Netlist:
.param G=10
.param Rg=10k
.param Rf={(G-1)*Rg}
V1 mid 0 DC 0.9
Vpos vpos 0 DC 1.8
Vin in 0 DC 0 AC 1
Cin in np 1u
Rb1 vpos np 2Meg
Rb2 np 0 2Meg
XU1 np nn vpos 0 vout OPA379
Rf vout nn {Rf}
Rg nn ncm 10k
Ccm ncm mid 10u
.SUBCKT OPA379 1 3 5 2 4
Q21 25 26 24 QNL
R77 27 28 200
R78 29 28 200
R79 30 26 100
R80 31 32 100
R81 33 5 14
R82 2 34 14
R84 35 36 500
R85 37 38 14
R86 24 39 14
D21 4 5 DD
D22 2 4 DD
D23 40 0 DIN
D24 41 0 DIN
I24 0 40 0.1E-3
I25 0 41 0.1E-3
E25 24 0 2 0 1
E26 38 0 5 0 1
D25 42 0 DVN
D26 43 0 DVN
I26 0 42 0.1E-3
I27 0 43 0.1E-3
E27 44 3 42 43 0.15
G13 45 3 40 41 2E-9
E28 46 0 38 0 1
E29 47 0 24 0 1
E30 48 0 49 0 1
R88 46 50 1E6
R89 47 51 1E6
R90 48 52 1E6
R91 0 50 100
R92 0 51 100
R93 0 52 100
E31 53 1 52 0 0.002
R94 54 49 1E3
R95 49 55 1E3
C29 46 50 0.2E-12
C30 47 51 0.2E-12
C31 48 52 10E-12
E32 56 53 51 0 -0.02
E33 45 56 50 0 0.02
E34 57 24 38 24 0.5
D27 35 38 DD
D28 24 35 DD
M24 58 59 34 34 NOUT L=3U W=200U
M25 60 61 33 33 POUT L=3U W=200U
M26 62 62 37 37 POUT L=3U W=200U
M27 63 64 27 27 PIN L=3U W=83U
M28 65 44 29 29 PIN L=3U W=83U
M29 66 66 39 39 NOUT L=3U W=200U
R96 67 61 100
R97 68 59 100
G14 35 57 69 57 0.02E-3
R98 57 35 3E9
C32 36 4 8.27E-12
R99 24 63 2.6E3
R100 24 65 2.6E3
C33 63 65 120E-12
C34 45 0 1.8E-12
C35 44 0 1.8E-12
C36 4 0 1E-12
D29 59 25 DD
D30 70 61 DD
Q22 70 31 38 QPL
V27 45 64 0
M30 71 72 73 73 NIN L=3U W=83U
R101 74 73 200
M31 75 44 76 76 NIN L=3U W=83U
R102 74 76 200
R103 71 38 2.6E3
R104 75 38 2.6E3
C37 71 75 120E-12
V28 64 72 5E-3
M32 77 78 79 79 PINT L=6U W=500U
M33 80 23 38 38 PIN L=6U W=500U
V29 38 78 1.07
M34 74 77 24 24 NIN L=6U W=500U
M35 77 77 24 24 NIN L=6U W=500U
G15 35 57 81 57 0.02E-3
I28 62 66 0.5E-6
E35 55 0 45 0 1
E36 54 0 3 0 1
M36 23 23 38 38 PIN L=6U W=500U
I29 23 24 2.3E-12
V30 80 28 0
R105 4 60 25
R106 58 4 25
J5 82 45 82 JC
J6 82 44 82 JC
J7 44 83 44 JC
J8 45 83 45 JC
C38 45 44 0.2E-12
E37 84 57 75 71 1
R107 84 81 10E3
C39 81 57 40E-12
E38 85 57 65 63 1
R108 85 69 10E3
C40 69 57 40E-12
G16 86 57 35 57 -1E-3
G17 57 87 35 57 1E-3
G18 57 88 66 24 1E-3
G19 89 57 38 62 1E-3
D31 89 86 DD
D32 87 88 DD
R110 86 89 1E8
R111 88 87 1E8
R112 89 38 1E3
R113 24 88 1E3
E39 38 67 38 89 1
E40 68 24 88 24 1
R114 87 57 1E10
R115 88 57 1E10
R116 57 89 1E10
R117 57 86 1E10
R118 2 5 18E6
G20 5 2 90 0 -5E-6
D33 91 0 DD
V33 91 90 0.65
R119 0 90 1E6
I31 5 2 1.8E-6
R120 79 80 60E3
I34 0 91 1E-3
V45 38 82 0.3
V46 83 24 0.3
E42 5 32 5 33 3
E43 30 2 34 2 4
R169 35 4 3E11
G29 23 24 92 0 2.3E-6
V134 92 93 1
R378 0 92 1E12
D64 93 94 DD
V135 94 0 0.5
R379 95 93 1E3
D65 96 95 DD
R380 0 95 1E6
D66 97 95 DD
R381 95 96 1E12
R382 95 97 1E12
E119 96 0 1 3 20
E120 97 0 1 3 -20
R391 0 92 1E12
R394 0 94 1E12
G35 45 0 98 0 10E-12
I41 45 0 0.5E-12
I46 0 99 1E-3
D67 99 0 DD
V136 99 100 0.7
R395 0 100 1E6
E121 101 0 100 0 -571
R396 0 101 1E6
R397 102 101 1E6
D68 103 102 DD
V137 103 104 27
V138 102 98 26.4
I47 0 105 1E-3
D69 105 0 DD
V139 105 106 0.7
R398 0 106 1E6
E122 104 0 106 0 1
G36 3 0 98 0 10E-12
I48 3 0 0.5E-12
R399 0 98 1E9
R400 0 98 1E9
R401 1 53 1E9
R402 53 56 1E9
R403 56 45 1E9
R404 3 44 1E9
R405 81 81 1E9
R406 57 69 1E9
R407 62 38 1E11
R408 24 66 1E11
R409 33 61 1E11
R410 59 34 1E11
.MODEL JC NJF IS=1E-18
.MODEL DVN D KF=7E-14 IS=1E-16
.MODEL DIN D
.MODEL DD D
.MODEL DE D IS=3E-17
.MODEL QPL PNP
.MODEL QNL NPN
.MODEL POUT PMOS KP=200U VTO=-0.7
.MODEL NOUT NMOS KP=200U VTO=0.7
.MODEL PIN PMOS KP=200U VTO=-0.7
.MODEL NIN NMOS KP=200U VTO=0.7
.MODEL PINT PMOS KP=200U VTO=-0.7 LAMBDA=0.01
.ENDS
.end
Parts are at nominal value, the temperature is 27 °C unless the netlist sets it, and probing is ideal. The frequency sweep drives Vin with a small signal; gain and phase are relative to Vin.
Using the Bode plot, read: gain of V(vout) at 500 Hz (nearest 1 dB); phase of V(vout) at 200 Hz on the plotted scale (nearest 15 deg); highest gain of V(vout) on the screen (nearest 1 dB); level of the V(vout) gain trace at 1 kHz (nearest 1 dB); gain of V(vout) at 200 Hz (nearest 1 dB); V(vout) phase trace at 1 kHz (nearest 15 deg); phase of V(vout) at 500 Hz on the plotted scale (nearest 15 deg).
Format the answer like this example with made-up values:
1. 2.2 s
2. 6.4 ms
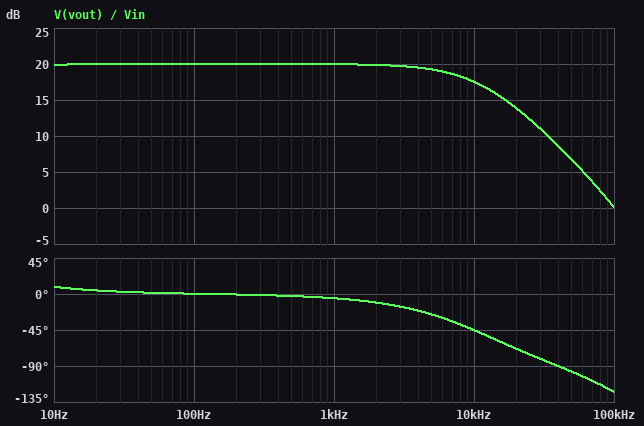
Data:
1. 20 dB
2. 0 deg
3. 20 dB
4. 20 dB
5. 20 dB
6. 0 deg
7. 0 deg
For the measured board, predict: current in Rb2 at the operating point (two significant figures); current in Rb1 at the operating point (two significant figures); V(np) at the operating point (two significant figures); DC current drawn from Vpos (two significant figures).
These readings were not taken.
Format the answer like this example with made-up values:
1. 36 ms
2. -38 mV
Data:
1. 450 nA
2. 450 nA
3. 900 mV
4. 2.8 µA
